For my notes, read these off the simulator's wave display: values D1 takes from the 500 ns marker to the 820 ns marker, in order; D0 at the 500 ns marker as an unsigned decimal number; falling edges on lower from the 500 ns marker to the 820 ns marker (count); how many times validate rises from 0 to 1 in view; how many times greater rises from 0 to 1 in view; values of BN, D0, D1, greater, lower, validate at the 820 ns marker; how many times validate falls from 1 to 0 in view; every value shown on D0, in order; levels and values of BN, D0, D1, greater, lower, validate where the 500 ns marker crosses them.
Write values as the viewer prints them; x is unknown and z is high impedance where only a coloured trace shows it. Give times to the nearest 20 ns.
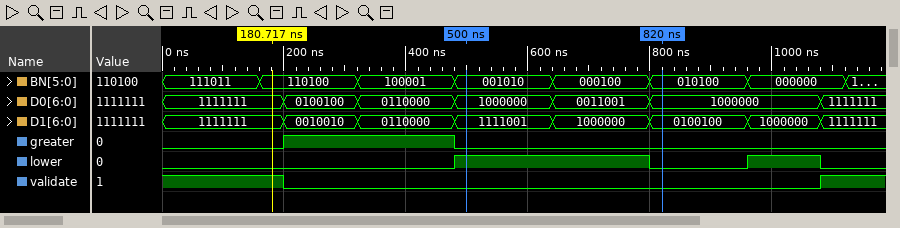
1111001, 1000000, 0100100
64
1
1
1
BN=010100, D0=1000000, D1=0100100, greater=0, lower=0, validate=0
1
1111111, 0100100, 0110000, 1000000, 0011001, 1000000, 1111111
BN=001010, D0=1000000, D1=1111001, greater=0, lower=1, validate=0
